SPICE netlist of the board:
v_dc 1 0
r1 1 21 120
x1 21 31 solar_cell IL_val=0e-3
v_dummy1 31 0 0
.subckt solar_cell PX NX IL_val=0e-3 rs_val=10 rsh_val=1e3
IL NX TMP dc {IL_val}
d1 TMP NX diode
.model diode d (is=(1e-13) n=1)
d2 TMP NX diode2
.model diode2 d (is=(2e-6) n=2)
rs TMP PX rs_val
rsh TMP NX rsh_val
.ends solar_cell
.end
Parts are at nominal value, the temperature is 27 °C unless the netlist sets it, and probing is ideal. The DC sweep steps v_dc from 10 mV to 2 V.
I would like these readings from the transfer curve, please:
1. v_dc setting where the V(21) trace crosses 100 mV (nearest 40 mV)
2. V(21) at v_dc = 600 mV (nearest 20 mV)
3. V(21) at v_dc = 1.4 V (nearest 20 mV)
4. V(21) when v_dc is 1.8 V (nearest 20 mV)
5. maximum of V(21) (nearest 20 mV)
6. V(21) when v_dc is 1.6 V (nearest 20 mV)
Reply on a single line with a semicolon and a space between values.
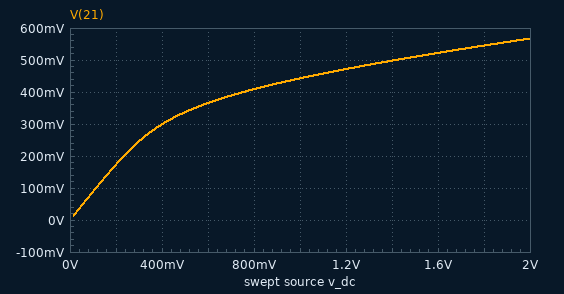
120 mV; 360 mV; 500 mV; 540 mV; 560 mV; 520 mV
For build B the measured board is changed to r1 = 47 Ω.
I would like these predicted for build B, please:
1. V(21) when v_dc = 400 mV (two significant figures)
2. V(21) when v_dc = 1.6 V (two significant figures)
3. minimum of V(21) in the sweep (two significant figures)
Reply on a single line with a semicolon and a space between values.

340 mV; 670 mV; 9.5 mV
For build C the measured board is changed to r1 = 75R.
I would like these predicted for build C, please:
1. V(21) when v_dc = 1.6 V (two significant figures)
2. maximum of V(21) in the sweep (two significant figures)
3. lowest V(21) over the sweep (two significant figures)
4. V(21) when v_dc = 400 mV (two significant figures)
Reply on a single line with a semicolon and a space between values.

590 mV; 650 mV; 9.3 mV; 320 mV
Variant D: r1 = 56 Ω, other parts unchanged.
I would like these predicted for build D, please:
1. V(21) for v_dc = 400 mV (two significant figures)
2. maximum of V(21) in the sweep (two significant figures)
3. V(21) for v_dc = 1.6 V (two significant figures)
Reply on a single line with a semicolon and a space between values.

330 mV; 710 mV; 640 mV
